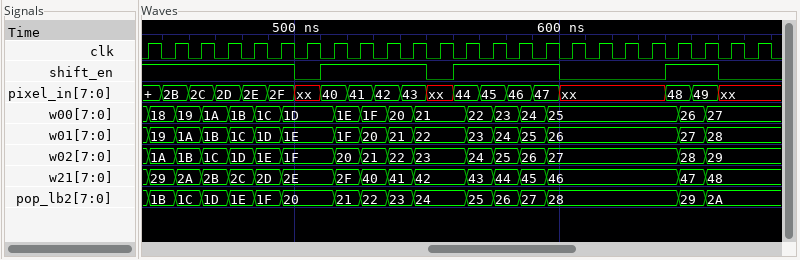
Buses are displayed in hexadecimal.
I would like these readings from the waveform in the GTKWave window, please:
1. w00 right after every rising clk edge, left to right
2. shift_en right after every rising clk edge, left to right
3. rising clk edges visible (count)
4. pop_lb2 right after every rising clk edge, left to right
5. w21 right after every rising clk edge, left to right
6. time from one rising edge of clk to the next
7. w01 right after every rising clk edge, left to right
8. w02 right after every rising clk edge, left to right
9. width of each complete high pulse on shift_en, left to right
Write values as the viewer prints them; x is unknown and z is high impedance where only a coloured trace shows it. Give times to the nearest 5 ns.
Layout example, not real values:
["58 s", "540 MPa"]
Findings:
["18, 19, 1A, 1B, 1C, 1D, 1D, 1E, 1F, 20, 21, 21, 22, 23, 24, 25, 25, 25, 25, 25, 26, 27, 27, 27", "1 1 1 1 1 1 0 1 1 1 1 0 1 1 1 1 0 0 0 0 1 1 0 0", "24", "1B, 1C, 1D, 1E, 1F, 20, 20, 21, 22, 23, 24, 24, 25, 26, 27, 28, 28, 28, 28, 28, 29, 2A, 2A, 2A", "29, 2A, 2B, 2C, 2D, 2E, 2E, 2F, 40, 41, 42, 42, 43, 44, 45, 46, 46, 46, 46, 46, 47, 48, 48, 48", "10 ns", "19, 1A, 1B, 1C, 1D, 1E, 1E, 1F, 20, 21, 22, 22, 23, 24, 25, 26, 26, 26, 26, 26, 27, 28, 28, 28", "1A, 1B, 1C, 1D, 1E, 1F, 1F, 20, 21, 22, 23, 23, 24, 25, 26, 27, 27, 27, 27, 27, 28, 29, 29, 29", "40 ns, 40 ns, 20 ns"]
